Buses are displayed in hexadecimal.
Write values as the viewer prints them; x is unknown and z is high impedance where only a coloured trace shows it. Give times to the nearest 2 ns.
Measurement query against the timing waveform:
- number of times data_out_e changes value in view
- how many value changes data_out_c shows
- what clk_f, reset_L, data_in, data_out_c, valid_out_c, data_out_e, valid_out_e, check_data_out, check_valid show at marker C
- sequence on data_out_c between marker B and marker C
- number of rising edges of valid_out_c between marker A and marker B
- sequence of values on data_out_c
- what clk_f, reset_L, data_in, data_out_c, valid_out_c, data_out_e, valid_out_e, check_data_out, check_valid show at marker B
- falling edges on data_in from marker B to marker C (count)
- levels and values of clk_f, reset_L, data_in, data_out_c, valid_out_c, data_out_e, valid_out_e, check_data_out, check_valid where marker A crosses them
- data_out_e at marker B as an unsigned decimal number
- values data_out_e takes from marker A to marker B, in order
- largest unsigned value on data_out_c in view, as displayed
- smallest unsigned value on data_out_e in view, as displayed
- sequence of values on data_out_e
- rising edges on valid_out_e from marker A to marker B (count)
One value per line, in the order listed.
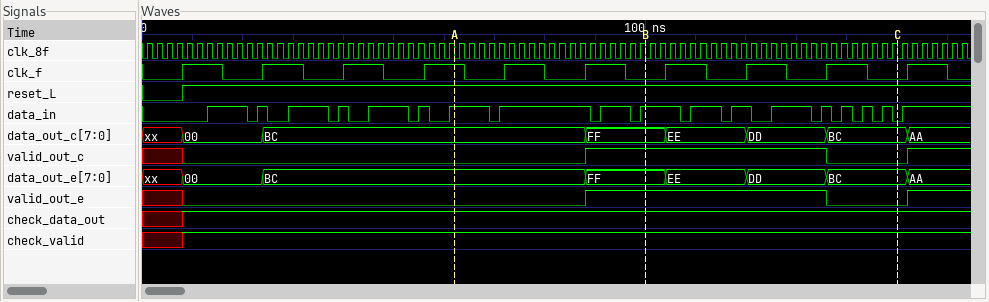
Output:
7
7
clk_f=0, reset_L=1, data_in=0, data_out_c=BC, valid_out_c=0, data_out_e=BC, valid_out_e=0, check_data_out=1, check_valid=1
FF, EE, DD, BC
1
xx, 00, BC, FF, EE, DD, BC, AA
clk_f=0, reset_L=1, data_in=1, data_out_c=FF, valid_out_c=1, data_out_e=FF, valid_out_e=1, check_data_out=1, check_valid=1
8
clk_f=1, reset_L=1, data_in=1, data_out_c=BC, valid_out_c=0, data_out_e=BC, valid_out_e=0, check_data_out=1, check_valid=1
255
BC, FF
FF
00
xx, 00, BC, FF, EE, DD, BC, AA
1
